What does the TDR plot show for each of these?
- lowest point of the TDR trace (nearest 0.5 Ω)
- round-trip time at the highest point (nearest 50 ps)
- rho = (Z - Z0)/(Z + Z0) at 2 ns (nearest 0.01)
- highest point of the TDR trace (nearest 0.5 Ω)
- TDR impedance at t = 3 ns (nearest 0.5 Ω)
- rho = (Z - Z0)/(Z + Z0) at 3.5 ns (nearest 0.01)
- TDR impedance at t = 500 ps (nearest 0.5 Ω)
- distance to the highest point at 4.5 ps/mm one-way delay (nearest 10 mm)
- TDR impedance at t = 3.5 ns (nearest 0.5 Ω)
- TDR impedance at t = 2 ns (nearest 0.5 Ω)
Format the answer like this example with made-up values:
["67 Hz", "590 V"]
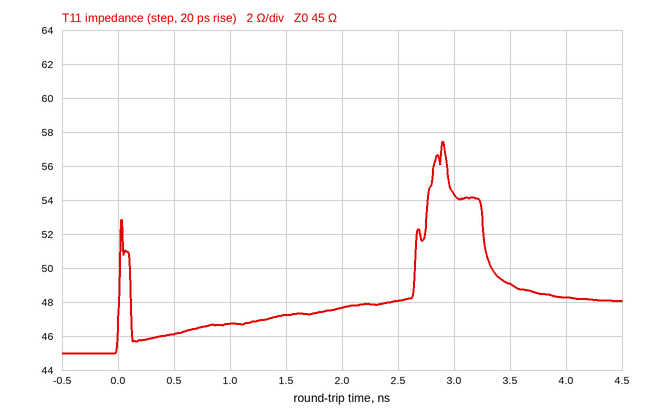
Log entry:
["45.0 Ω", "2.90 ns", "+0.03", "57.5 Ω", "54.5 Ω", "+0.04", "46.0 Ω", "320 mm", "49.0 Ω", "47.5 Ω"]
